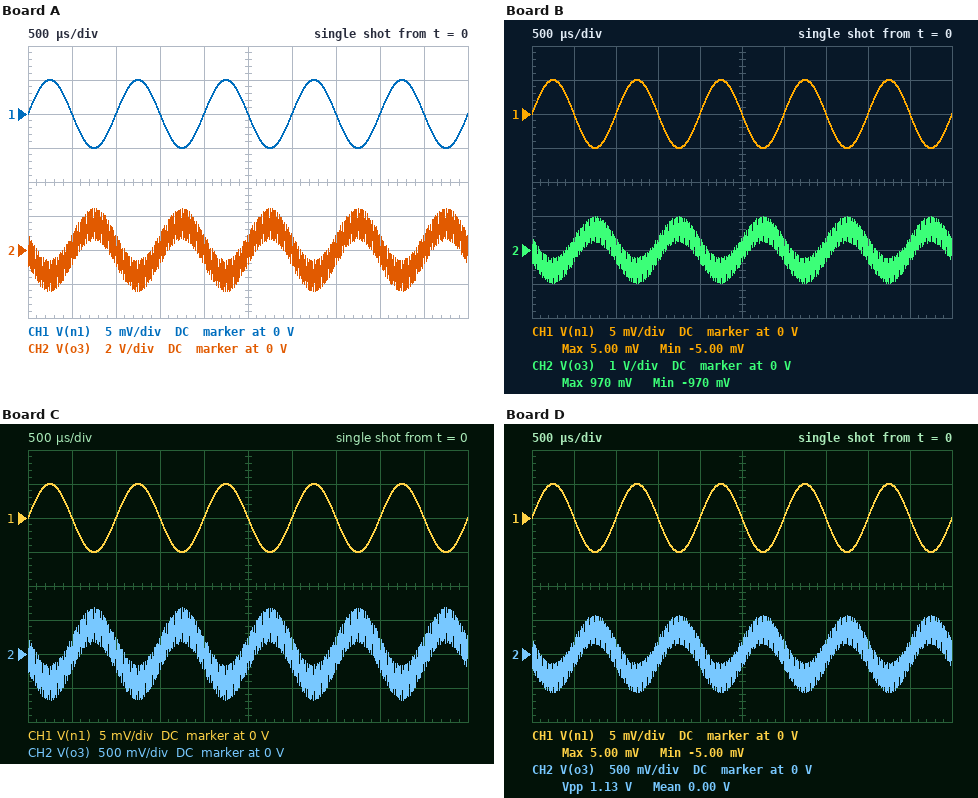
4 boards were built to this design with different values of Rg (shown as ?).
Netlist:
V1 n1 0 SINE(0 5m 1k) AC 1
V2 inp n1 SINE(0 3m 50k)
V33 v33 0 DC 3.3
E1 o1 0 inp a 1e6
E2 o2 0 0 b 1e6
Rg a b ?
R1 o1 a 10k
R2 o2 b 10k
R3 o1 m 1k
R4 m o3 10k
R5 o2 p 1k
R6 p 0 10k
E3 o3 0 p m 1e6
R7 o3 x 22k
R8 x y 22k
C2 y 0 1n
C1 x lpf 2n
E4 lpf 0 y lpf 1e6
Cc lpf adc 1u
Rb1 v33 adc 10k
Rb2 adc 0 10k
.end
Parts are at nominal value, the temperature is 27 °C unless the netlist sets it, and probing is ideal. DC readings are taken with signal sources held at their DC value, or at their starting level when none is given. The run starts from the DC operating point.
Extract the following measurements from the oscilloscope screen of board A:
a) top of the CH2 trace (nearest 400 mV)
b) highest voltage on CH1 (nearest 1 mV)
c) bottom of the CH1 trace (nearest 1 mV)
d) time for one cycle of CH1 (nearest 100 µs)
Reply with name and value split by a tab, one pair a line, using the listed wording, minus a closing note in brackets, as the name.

top of the CH2 trace	2.4 V
highest voltage on CH1	5 mV
bottom of the CH1 trace	-5 mV
time for one cycle of CH1	1.0 ms
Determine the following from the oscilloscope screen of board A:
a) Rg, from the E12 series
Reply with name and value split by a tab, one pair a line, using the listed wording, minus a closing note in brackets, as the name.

Rg, from the E12 series	680 Ω
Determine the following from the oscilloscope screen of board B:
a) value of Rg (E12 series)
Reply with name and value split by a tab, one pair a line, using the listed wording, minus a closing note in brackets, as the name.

value of Rg	1.8 kΩ
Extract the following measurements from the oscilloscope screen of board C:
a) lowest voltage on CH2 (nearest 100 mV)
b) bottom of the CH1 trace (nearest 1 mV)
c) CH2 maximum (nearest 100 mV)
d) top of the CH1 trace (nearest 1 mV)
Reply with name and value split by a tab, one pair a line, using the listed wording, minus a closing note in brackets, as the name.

lowest voltage on CH2	-700 mV
bottom of the CH1 trace	-5 mV
CH2 maximum	700 mV
top of the CH1 trace	5 mV
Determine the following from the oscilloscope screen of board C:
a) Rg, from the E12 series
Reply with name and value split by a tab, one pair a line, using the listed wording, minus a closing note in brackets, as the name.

Rg, from the E12 series	2.7 kΩ
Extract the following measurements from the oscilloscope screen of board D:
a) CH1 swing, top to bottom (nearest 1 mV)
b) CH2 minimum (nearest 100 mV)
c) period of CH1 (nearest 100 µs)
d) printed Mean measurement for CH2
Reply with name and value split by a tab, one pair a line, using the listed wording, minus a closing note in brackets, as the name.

CH1 swing, top to bottom	10 mV
CH2 minimum	-600 mV
period of CH1	1.0 ms
printed Mean measurement for CH2	0.00 V
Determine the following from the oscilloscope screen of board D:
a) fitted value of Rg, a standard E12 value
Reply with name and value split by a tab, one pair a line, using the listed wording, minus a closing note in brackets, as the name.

fitted value of Rg, a standard E12 value	3.3 kΩ
